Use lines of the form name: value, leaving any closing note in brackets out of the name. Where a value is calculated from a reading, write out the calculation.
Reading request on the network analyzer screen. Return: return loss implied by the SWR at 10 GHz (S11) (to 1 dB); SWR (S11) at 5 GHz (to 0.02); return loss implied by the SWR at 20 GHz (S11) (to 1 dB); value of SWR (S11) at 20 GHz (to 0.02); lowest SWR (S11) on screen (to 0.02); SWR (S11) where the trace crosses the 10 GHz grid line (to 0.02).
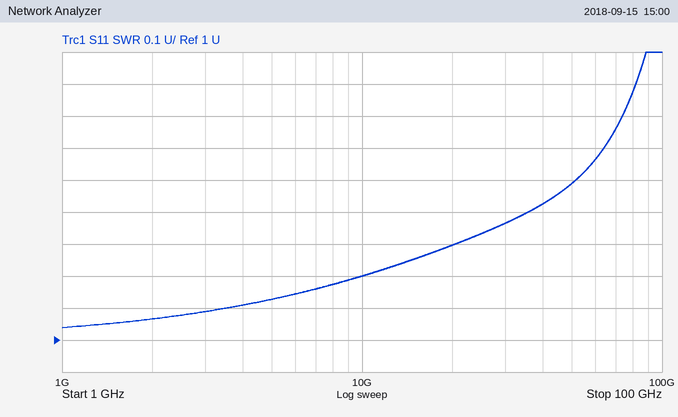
return loss implied by the SWR at 10 GHz (S11): −20 log10((1.2 − 1)/(1.2 + 1)) ≈ 21 dB
SWR (S11) at 5 GHz: 1.12
return loss implied by the SWR at 20 GHz (S11): −20 log10((1.3 − 1)/(1.3 + 1)) ≈ 18 dB
value of SWR (S11) at 20 GHz: 1.30
lowest SWR (S11) on screen: 1.04
SWR (S11) where the trace crosses the 10 GHz grid line: 1.20
